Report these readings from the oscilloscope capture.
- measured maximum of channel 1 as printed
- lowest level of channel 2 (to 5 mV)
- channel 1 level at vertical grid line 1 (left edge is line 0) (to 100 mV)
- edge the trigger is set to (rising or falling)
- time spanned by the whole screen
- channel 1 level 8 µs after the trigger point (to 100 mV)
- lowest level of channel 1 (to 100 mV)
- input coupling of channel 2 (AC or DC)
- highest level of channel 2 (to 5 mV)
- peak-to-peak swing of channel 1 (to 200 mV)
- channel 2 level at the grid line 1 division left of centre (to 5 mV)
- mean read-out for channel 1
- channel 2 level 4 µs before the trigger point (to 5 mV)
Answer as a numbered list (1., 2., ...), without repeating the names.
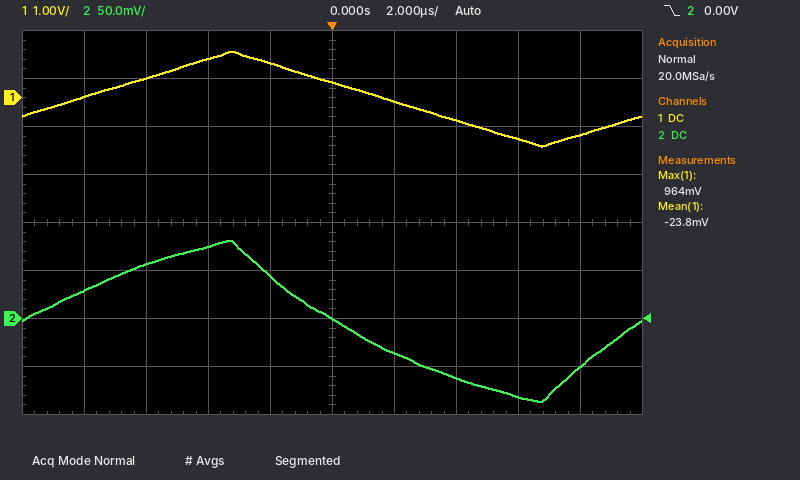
1. 964 mV
2. -85 mV
3. 0.0 V
4. falling
5. 20 µs
6. -800 mV
7. -1.0 V
8. DC
9. 80 mV
10. 2.0 V
11. 45 mV
12. -23.8 mV
13. 75 mV
